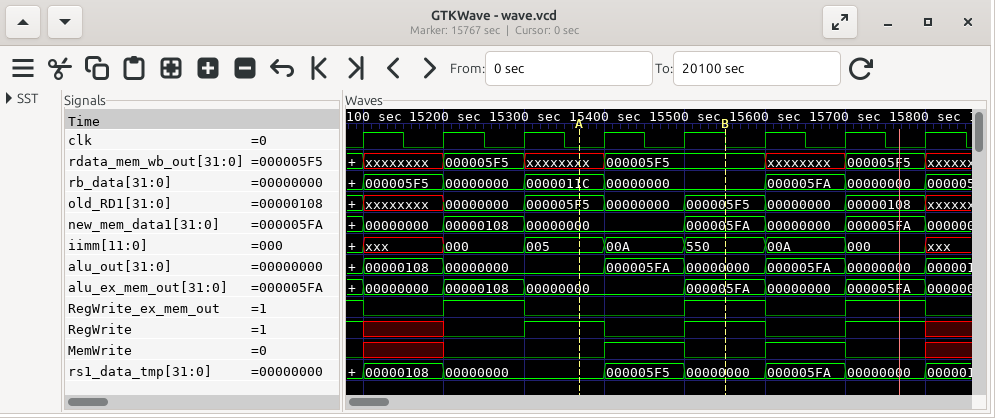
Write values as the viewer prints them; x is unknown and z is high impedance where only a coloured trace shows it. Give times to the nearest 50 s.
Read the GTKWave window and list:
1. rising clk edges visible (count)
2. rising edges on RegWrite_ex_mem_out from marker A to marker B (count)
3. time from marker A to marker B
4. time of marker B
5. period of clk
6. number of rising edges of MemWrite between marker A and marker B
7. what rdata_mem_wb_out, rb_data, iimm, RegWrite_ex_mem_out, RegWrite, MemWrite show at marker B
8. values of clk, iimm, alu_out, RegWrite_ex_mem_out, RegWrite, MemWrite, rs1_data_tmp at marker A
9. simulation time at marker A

8
1
200 s
15550 s
100 s
1
rdata_mem_wb_out=000005F5, rb_data=00000000, iimm=550, RegWrite_ex_mem_out=1, RegWrite=1, MemWrite=0
clk=0, iimm=005, alu_out=00000000, RegWrite_ex_mem_out=0, RegWrite=1, MemWrite=0, rs1_data_tmp=00000000
15350 s
